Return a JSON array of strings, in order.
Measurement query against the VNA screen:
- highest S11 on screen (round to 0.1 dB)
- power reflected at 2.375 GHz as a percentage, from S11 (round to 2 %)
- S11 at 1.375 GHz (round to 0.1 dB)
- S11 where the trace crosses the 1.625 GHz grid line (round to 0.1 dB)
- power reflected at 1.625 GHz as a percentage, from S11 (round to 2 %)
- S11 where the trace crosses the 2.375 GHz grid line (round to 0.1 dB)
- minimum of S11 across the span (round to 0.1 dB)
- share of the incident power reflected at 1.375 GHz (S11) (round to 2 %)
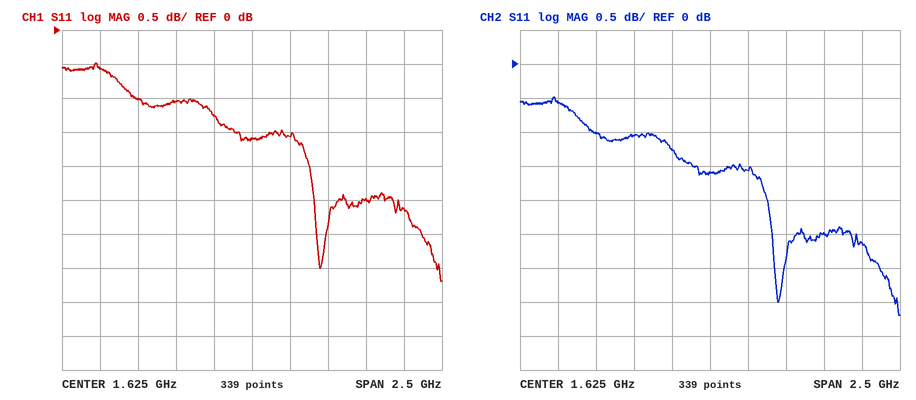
["-0.5 dB", "56 %", "-1.3 dB", "-1.6 dB", "70 %", "-2.5 dB", "-3.7 dB", "74 %"]
